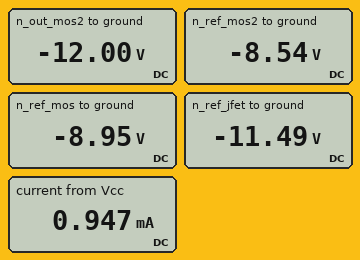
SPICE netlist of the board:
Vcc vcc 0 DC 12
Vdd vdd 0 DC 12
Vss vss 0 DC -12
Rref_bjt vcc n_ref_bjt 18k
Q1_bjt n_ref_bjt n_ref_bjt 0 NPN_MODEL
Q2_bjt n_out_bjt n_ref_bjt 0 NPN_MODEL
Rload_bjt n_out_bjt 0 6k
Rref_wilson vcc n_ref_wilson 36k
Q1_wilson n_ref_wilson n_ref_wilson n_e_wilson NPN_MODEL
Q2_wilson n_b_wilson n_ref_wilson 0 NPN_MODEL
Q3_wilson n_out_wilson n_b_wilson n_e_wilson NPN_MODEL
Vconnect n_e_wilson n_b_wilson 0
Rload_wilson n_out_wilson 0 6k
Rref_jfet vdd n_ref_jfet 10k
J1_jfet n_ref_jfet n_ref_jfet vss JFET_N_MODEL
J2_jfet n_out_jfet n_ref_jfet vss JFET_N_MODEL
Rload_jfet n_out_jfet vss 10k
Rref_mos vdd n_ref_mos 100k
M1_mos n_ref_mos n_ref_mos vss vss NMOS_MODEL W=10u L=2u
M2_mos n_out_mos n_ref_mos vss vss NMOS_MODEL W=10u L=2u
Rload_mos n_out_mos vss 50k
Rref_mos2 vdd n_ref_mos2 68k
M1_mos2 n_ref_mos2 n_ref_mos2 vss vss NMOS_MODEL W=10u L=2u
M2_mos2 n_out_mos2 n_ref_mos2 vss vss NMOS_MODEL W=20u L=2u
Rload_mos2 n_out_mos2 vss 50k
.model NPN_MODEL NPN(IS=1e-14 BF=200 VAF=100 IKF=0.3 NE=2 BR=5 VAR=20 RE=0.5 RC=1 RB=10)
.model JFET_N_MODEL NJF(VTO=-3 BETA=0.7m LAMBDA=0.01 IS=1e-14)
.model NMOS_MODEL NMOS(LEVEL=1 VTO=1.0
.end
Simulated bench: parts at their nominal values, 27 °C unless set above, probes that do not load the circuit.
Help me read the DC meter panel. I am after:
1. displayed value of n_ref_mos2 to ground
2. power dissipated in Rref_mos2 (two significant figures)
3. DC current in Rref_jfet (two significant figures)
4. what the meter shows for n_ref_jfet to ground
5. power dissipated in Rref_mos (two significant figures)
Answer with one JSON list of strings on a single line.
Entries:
["-8.54 V", "6.2 mW", "2.3 mA", "-11.49 V", "4.4 mW"]
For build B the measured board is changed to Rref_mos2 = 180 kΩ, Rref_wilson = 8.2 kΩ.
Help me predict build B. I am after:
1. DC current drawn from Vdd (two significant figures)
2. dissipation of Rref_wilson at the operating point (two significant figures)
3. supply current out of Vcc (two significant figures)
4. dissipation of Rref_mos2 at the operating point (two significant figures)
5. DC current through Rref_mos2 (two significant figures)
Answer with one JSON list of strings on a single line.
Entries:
["2.7 mA", "16 mW", "2.0 mA", "2.6 mW", "120 µA"]
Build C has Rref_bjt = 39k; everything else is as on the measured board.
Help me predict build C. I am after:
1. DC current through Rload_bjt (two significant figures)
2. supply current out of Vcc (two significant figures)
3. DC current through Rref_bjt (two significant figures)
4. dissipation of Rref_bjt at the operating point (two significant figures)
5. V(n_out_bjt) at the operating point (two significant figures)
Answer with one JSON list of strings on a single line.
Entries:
["800 nA", "610 µA", "290 µA", "3.3 mW", "4.8 mV"]
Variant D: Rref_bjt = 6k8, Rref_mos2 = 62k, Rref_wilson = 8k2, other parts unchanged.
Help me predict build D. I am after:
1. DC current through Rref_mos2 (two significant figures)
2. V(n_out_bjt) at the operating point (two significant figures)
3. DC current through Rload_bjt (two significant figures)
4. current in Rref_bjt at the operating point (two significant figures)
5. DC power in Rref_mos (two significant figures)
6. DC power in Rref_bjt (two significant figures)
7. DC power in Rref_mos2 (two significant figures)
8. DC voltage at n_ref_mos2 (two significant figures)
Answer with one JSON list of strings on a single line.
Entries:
["330 µA", "5.0 mV", "840 nA", "1.7 mA", "4.4 mW", "19 mW", "6.7 mW", "-8.4 V"]
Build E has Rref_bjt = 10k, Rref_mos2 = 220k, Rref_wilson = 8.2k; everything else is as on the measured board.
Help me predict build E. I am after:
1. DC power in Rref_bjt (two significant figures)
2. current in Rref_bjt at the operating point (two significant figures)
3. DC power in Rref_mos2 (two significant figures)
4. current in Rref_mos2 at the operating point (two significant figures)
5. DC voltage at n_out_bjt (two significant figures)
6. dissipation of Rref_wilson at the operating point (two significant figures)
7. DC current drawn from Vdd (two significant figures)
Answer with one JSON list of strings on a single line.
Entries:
["13 mW", "1.1 mA", "2.1 mW", "98 µA", "5.0 mV", "16 mW", "2.7 mA"]
